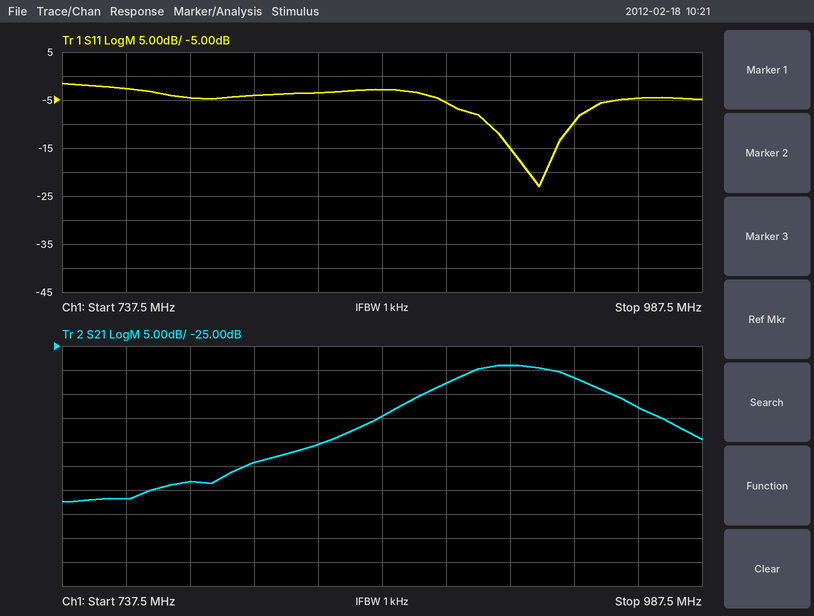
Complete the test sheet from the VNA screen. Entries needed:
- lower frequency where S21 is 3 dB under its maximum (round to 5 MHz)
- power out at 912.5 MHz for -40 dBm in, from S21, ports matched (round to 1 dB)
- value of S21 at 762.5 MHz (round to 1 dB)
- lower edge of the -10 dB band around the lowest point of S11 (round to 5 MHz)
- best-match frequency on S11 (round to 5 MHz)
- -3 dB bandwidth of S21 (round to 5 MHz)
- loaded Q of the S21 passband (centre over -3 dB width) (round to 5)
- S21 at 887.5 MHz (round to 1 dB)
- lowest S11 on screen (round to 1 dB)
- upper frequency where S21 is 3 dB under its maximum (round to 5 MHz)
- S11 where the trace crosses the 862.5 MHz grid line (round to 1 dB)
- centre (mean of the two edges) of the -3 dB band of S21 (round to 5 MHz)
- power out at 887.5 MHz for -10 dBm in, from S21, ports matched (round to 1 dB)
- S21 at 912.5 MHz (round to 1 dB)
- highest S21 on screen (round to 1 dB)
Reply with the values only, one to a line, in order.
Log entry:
890 MHz
-69 dBm
-57 dB
905 MHz
925 MHz
50 MHz
20
-33 dB
-23 dB
940 MHz
-3 dB
915 MHz
-43 dBm
-29 dB
-29 dB
